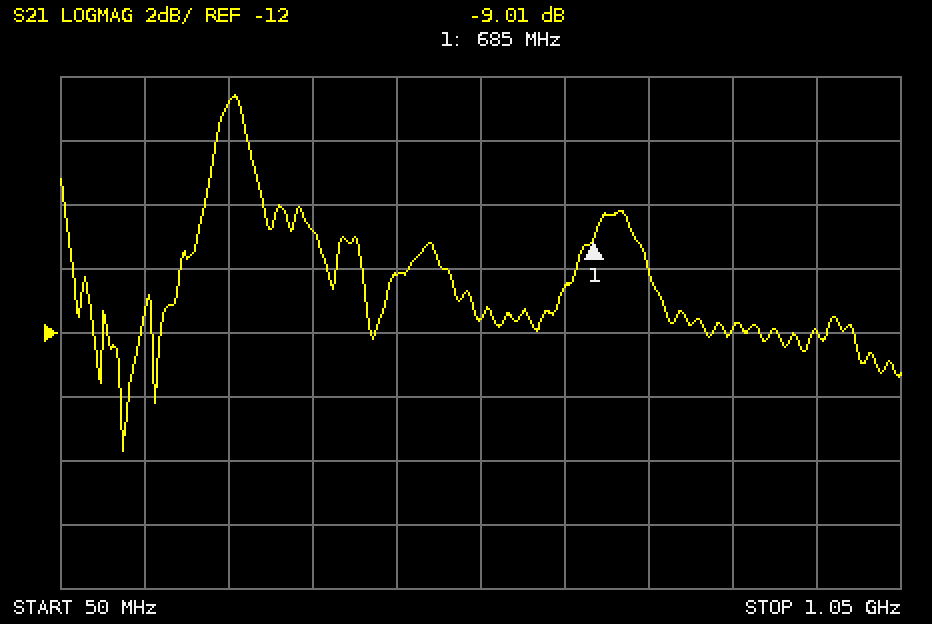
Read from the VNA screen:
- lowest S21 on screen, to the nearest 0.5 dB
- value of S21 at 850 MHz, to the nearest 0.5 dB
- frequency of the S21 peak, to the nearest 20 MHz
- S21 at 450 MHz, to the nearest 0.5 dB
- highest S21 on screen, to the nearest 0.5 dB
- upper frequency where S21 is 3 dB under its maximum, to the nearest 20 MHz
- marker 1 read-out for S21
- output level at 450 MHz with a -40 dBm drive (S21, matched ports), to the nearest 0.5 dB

-15.5 dB
-12.0 dB
260 MHz
-10.0 dB
-4.5 dB
280 MHz
-9.01 dB
-50.0 dBm
